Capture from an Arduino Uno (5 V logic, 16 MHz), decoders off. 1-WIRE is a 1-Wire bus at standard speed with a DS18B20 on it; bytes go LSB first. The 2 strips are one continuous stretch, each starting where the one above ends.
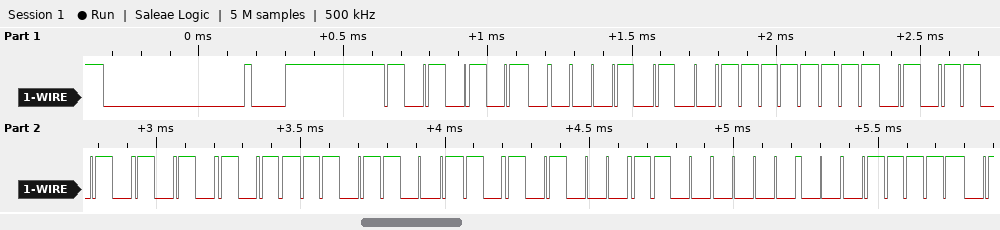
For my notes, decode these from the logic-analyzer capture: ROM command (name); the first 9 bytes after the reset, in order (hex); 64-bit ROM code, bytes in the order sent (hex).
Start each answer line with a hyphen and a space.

- Match ROM
- 55 28 FF 5A D5 9B 15 03 F8
- 28 FF 5A D5 9B 15 03 F8
